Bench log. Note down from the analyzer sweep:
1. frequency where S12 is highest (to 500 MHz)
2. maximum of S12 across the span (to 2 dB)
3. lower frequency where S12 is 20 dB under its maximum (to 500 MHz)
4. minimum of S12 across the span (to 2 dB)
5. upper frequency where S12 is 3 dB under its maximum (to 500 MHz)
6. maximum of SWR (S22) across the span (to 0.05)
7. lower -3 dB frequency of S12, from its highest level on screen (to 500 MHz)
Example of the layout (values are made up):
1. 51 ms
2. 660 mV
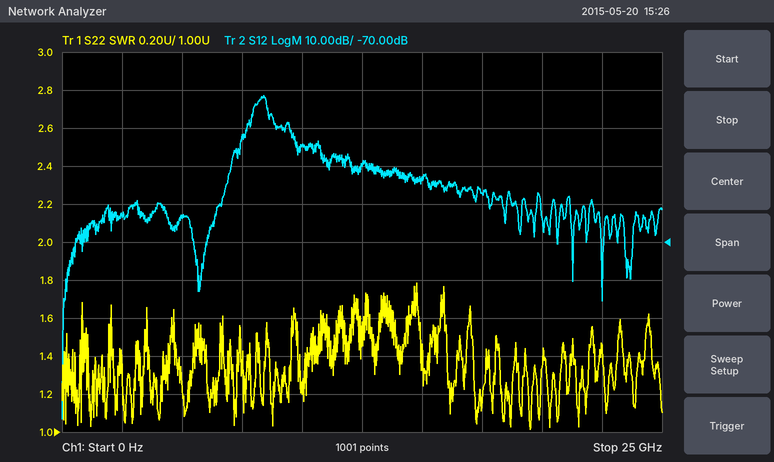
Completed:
1. 8.5 GHz
2. -32 dB
3. 7.0 GHz
4. -116 dB
5. 8.5 GHz
6. 1.80
7. 8.0 GHz
